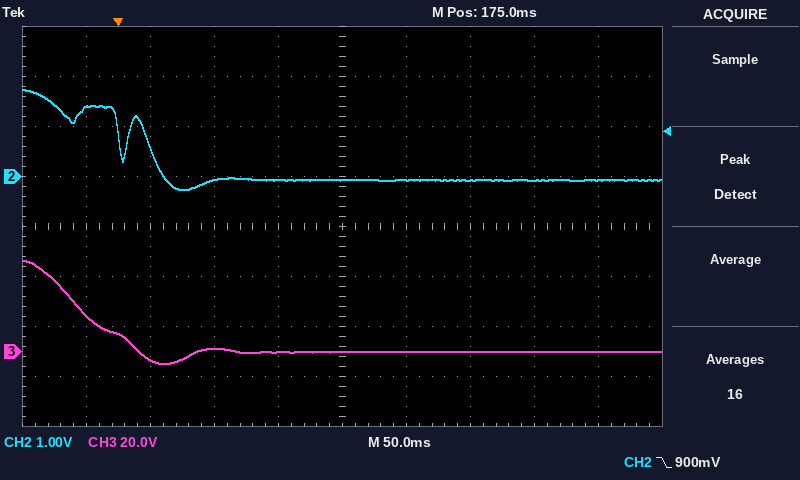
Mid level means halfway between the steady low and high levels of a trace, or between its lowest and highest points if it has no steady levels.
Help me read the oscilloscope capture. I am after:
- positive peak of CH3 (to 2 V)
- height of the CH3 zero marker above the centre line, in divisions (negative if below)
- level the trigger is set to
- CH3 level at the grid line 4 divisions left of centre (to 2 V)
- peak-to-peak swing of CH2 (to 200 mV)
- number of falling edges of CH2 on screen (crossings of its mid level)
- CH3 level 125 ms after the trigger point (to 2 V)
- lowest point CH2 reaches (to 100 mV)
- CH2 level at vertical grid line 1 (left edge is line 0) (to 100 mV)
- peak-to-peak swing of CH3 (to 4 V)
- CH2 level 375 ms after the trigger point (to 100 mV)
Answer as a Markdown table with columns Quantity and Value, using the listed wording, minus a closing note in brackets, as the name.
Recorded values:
| Quantity | Value |
|---|---|
| positive peak of CH3 | 36 V |
| height of the CH3 zero marker above the centre line, in divisions | -2.5 div |
| level the trigger is set to | 900 mV |
| CH3 level at the grid line 4 divisions left of centre | 14 V |
| peak-to-peak swing of CH2 | 2.0 V |
| number of falling edges of CH2 on screen | 2 |
| CH3 level 125 ms after the trigger point | 0 V |
| lowest point CH2 reaches | -300 mV |
| CH2 level at vertical grid line 1 (left edge is line 0) | 1.4 V |
| peak-to-peak swing of CH3 | 40 V |
| CH2 level 375 ms after the trigger point | -100 mV |
